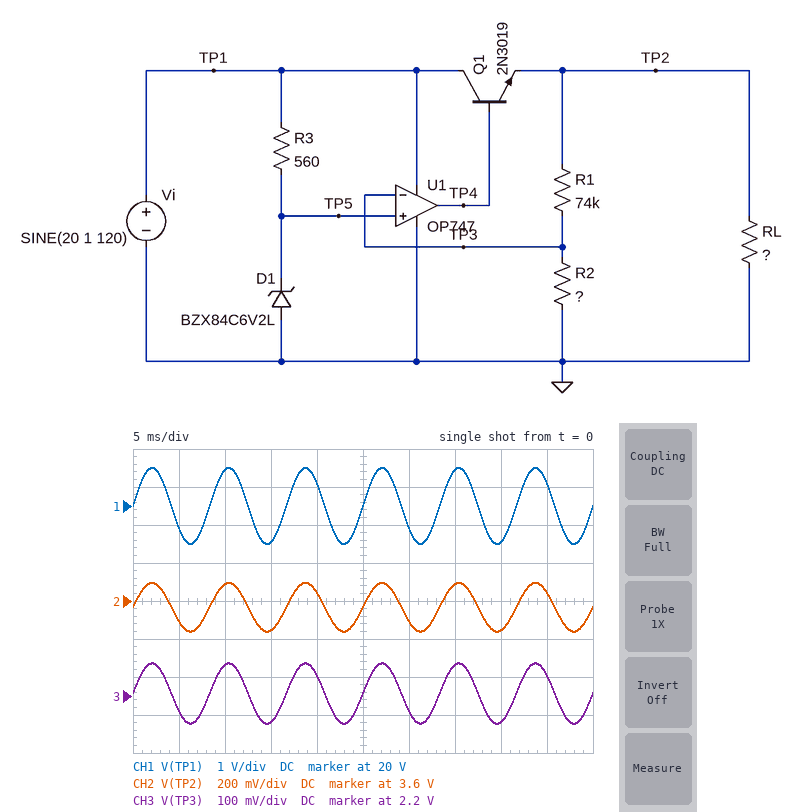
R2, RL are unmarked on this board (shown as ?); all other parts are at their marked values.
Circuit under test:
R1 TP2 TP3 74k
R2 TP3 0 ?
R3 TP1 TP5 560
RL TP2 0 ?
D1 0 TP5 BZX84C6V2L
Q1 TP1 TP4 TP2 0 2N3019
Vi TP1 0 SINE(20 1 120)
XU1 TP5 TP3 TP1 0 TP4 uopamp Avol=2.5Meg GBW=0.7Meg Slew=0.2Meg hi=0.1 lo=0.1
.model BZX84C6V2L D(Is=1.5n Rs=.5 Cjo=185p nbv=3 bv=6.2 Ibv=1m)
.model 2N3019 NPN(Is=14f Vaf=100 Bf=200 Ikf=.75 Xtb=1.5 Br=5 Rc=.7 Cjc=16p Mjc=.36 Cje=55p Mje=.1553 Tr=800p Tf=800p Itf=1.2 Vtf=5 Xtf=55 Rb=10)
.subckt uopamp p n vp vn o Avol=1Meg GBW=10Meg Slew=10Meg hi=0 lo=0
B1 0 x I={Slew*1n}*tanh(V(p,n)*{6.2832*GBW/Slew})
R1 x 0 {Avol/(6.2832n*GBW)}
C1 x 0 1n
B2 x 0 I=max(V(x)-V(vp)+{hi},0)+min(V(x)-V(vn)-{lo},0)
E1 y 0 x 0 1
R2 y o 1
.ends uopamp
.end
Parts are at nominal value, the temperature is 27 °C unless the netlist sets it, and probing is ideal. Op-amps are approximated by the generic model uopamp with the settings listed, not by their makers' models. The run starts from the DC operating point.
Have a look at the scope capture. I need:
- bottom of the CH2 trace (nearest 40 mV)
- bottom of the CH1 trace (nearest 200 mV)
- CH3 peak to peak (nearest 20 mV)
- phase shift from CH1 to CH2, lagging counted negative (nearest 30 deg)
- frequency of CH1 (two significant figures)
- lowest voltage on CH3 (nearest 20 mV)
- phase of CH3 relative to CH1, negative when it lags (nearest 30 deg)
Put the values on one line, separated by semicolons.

3.44 V; 19.0 V; 160 mV; 0 deg; 120 Hz; 2.12 V; 0 deg
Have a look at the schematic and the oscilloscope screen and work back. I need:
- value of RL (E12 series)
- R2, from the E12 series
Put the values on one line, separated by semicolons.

0.22 Ω; 120 kΩ
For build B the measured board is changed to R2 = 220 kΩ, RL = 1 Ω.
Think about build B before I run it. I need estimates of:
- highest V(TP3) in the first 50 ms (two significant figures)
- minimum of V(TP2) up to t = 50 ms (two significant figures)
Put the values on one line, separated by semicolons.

6.5 V; 8.6 V
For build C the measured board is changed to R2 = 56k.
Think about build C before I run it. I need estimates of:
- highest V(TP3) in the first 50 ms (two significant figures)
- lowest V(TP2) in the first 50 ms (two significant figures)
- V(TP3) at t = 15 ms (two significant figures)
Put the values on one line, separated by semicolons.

1.6 V; 3.4 V; 1.5 V
